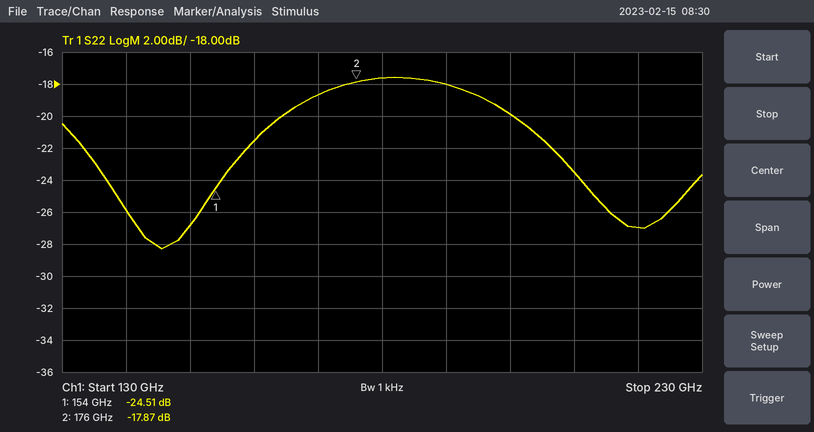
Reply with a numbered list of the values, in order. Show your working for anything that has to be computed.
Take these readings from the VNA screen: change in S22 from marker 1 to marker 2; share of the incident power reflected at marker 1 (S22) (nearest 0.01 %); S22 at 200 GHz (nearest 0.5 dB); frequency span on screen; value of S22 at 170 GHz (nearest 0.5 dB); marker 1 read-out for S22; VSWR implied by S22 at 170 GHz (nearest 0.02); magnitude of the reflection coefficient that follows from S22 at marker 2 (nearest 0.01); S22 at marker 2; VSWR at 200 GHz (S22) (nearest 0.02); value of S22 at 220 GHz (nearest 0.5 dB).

1. -17.87 − (-24.51) = 6.64 dB
2. 10^(-24.51/10) ≈ 0.35 %
3. -20.0 dB
4. 100 GHz
5. -18.5 dB
6. -24.51 dB
7. |Γ| = 10^(-18.5/20) = 0.1189; VSWR = (1 + 0.1189)/(1 − 0.1189) ≈ 1.27, so 1.26 to the nearest 0.02
8. 10^(-17.87/20) ≈ 0.13
9. -17.87 dB
10. |Γ| = 10^(-20/20) = 0.1000; VSWR = (1 + 0.1000)/(1 − 0.1000) ≈ 1.22
11. -27.0 dB
